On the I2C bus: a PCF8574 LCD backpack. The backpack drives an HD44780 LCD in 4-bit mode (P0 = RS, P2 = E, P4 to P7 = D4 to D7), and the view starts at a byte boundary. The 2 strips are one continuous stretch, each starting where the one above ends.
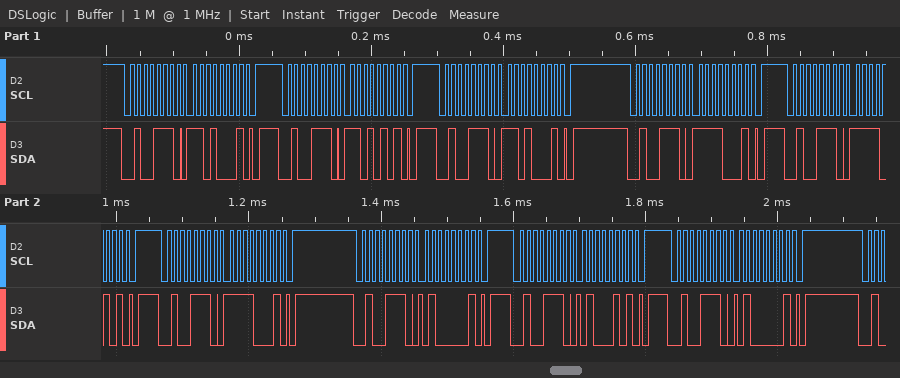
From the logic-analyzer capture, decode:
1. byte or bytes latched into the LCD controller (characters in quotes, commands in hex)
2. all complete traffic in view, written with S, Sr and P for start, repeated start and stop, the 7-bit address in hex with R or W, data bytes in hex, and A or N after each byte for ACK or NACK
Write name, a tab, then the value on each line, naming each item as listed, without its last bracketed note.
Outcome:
byte or bytes latched into the LCD controller	data 0xDF
all complete traffic in view, written with S, Sr and P for start, repeated start and stop, the 7-bit address in hex with R or W, data bytes in hex, and A or N after each byte for ACK or NACK	S 27W A D1 A P S 27W A D5 A P S 27W A D1 A P S 27W A F1 A P S 27W A F5 A P S 27W A F1 A P S 27W A 41 A P S 27W A 45 A P S 27W A 41 A P
